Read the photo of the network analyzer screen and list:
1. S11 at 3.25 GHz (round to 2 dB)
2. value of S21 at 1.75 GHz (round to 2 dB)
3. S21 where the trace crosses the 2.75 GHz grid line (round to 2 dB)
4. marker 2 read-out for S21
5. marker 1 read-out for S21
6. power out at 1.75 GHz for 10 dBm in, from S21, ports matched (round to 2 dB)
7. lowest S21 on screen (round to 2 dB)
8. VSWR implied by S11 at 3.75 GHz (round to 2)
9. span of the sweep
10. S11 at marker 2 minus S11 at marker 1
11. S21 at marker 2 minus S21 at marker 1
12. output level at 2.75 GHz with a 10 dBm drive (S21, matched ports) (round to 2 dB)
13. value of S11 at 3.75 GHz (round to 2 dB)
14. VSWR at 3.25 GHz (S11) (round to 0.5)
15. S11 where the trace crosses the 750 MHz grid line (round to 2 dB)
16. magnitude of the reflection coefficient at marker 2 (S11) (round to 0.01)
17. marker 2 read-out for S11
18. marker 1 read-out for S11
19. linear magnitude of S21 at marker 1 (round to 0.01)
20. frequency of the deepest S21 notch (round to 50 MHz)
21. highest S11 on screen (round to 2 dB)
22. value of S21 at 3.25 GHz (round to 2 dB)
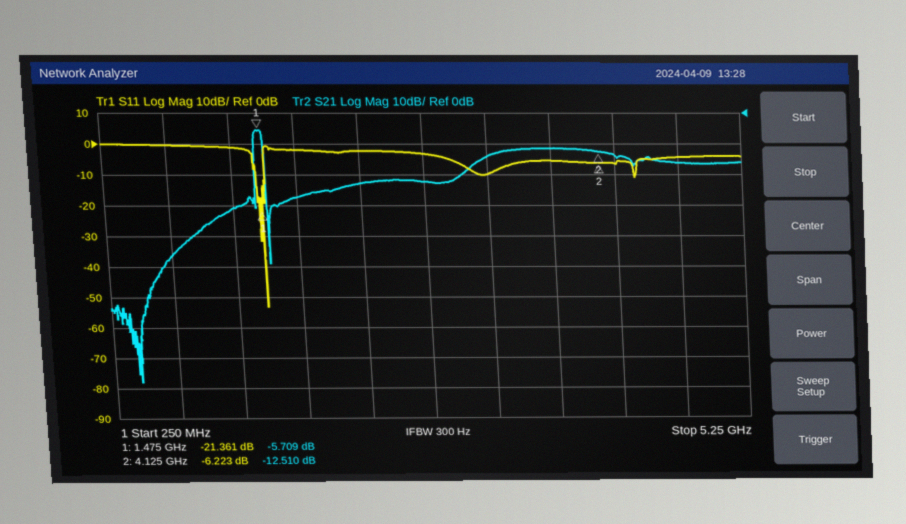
-10 dB
-28 dB
-22 dB
-12.510 dB
-5.709 dB
-18 dBm
-88 dB
4
5 GHz
15.138 dB
-6.801 dB
-12 dBm
-6 dB
2.0
0 dB
0.49
-6.223 dB
-21.361 dB
0.52
450 MHz
0 dB
-14 dB
